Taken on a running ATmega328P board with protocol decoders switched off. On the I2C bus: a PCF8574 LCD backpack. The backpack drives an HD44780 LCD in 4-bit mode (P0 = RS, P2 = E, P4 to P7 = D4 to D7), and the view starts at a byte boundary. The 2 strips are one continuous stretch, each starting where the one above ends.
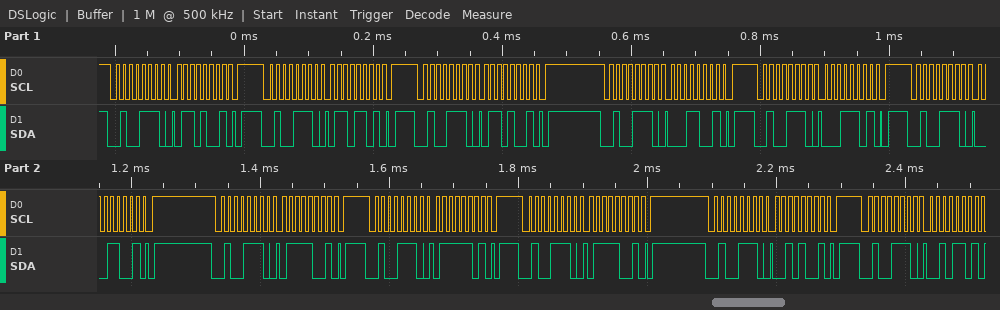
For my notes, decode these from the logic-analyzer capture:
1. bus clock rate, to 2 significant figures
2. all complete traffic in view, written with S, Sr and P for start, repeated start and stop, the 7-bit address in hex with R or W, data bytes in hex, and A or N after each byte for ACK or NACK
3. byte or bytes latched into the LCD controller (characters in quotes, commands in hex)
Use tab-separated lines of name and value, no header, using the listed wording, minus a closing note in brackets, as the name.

bus clock rate, to 2 significant figures	100 kHz
all complete traffic in view, written with S, Sr and P for start, repeated start and stop, the 7-bit address in hex with R or W, data bytes in hex, and A or N after each byte for ACK or NACK	S 27W A 69 A P S 27W A 6D A P S 27W A 69 A P S 27W A 19 A P S 27W A 1D A P S 27W A 19 A P S 27W A 79 A P S 27W A 7D A P S 27W A 79 A P S 27W A 29 A P S 27W A 2D A
byte or bytes latched into the LCD controller	'a'
